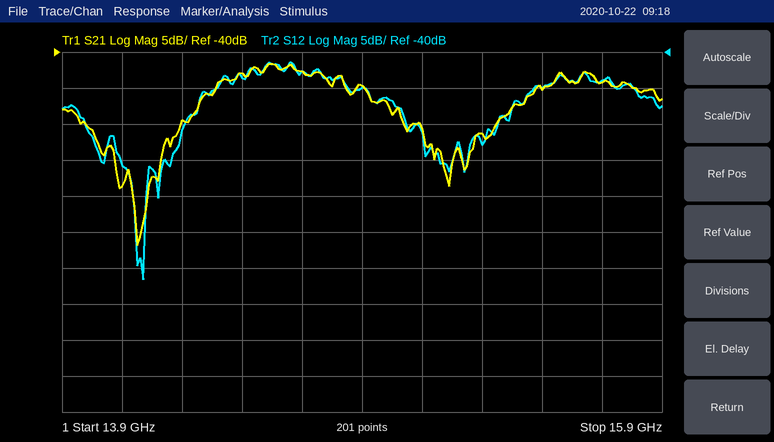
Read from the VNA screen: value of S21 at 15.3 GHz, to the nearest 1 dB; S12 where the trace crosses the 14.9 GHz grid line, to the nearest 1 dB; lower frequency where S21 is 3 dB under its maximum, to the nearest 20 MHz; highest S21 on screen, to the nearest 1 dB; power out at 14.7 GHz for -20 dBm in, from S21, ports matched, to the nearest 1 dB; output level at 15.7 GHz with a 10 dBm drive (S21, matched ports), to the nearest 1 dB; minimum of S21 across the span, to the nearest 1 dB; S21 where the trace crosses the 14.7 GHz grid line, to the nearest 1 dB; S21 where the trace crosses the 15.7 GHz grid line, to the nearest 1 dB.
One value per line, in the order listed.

-51 dB
-45 dB
14.42 GHz
-42 dB
-63 dBm
-34 dBm
-67 dB
-43 dB
-44 dB
